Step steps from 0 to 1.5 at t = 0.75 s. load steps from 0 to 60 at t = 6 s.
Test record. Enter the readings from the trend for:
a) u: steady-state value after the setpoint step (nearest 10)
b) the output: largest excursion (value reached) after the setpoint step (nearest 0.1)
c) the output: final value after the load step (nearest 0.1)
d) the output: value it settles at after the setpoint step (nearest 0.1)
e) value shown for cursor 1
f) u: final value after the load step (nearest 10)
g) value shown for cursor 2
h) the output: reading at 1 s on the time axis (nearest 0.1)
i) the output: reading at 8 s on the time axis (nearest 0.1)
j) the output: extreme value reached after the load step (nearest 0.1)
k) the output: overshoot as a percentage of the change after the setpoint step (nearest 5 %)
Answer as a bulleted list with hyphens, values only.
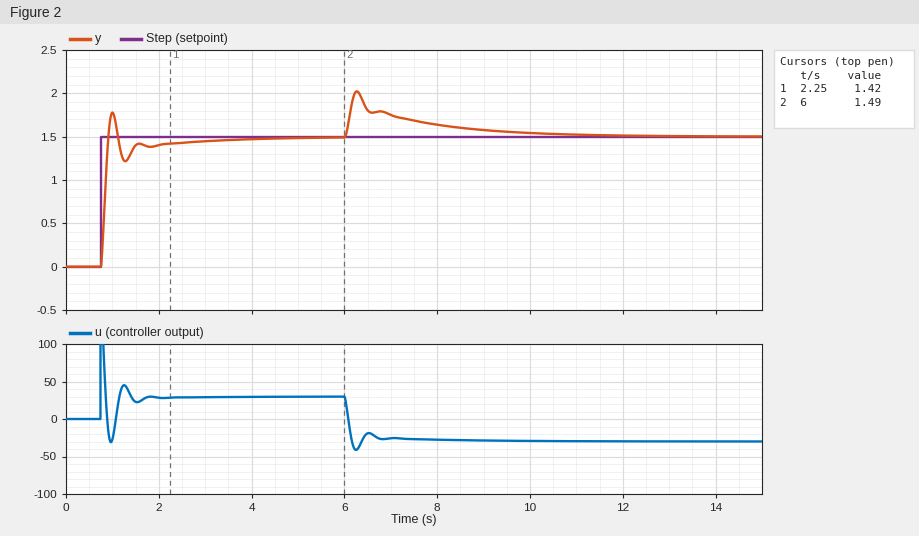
- 30
- 1.8
- 1.5
- 1.5
- 1.42
- -30
- 1.49
- 1.8
- 1.6
- 2.0
- 20 %
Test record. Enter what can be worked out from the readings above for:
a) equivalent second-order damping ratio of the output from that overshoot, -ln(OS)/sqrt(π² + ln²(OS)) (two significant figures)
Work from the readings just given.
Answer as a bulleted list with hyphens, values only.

- 0.46
